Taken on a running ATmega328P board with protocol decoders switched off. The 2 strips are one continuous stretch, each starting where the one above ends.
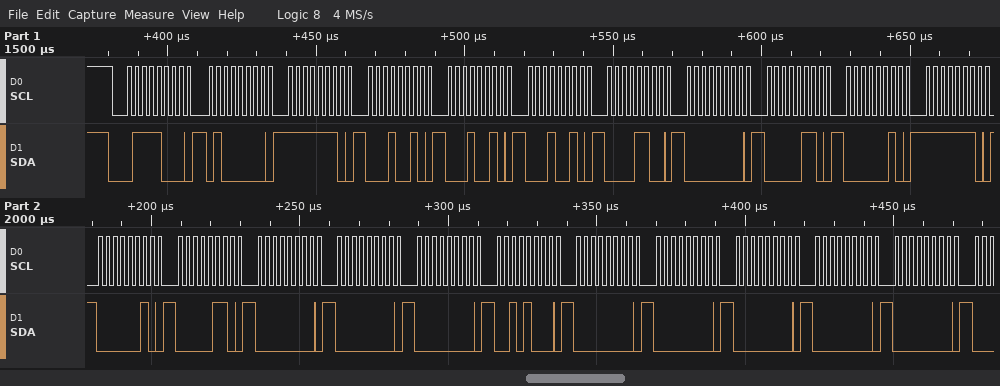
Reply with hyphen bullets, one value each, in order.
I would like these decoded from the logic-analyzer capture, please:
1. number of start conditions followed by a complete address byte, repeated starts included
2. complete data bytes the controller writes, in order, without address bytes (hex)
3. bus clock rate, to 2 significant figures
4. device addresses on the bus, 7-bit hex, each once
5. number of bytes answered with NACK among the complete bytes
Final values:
- 1
- 40 FE 12 12 12 0C 00 06 02 FE 02 06 00 00 00 28 00 00 00 00 00
- 400 kHz
- 0x3C
- 0
